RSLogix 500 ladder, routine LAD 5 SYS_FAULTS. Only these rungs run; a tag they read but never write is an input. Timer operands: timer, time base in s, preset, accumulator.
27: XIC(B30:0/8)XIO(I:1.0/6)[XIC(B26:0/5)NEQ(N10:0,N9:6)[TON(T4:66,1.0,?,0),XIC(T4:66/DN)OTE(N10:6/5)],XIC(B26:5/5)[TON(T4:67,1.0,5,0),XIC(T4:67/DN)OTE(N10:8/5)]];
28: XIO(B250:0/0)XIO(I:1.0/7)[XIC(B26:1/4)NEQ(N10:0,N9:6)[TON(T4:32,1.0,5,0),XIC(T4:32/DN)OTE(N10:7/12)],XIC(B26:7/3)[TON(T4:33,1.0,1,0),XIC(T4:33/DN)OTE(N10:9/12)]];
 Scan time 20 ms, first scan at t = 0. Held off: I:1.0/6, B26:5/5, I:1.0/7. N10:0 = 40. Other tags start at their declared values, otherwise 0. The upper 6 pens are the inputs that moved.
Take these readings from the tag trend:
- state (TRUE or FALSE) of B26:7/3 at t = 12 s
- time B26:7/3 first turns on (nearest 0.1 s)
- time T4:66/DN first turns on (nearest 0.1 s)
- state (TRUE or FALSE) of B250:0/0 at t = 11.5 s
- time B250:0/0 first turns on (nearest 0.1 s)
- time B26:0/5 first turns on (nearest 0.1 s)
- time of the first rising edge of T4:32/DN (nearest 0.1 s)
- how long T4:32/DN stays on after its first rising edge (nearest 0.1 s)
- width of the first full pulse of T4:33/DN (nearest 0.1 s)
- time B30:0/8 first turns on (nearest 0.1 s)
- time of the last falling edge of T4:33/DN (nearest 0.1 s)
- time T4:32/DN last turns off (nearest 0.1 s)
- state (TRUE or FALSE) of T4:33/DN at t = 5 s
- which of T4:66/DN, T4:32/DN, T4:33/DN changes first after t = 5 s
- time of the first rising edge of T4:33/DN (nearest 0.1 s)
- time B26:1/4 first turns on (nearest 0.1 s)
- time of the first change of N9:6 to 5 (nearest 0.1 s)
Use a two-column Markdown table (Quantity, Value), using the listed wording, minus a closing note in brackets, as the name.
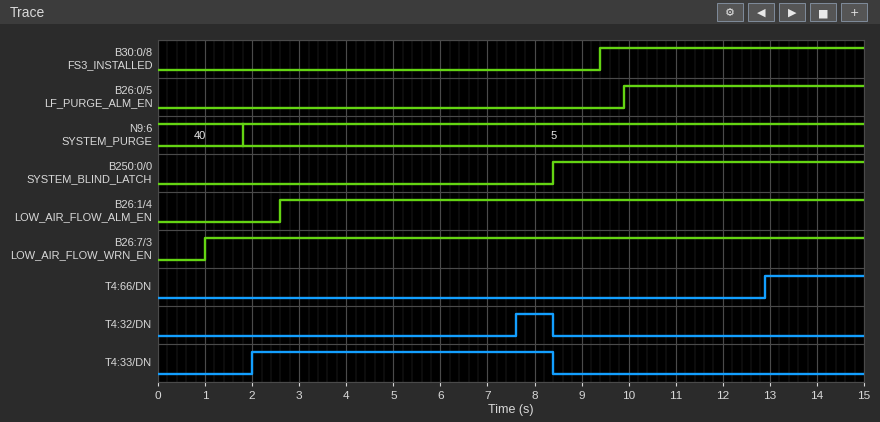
| Quantity | Value |
|---|---|
| state (TRUE or FALSE) of B26:7/3 at t = 12 s | TRUE |
| time B26:7/3 first turns on | 1.0 s |
| time T4:66/DN first turns on | 12.9 s |
| state (TRUE or FALSE) of B250:0/0 at t = 11.5 s | TRUE |
| time B250:0/0 first turns on | 8.4 s |
| time B26:0/5 first turns on | 9.9 s |
| time of the first rising edge of T4:32/DN | 7.6 s |
| how long T4:32/DN stays on after its first rising edge | 0.8 s |
| width of the first full pulse of T4:33/DN | 6.4 s |
| time B30:0/8 first turns on | 9.4 s |
| time of the last falling edge of T4:33/DN | 8.4 s |
| time T4:32/DN last turns off | 8.4 s |
| state (TRUE or FALSE) of T4:33/DN at t = 5 s | TRUE |
| which of T4:66/DN, T4:32/DN, T4:33/DN changes first after t = 5 s | T4:32/DN |
| time of the first rising edge of T4:33/DN | 2.0 s |
| time B26:1/4 first turns on | 2.6 s |
| time of the first change of N9:6 to 5 | 1.8 s |
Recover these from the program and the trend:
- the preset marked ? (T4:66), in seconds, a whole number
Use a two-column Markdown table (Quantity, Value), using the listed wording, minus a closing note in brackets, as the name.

| Quantity | Value |
|---|---|
| the preset marked ? (T4:66), in seconds, a whole number | 3 s |
